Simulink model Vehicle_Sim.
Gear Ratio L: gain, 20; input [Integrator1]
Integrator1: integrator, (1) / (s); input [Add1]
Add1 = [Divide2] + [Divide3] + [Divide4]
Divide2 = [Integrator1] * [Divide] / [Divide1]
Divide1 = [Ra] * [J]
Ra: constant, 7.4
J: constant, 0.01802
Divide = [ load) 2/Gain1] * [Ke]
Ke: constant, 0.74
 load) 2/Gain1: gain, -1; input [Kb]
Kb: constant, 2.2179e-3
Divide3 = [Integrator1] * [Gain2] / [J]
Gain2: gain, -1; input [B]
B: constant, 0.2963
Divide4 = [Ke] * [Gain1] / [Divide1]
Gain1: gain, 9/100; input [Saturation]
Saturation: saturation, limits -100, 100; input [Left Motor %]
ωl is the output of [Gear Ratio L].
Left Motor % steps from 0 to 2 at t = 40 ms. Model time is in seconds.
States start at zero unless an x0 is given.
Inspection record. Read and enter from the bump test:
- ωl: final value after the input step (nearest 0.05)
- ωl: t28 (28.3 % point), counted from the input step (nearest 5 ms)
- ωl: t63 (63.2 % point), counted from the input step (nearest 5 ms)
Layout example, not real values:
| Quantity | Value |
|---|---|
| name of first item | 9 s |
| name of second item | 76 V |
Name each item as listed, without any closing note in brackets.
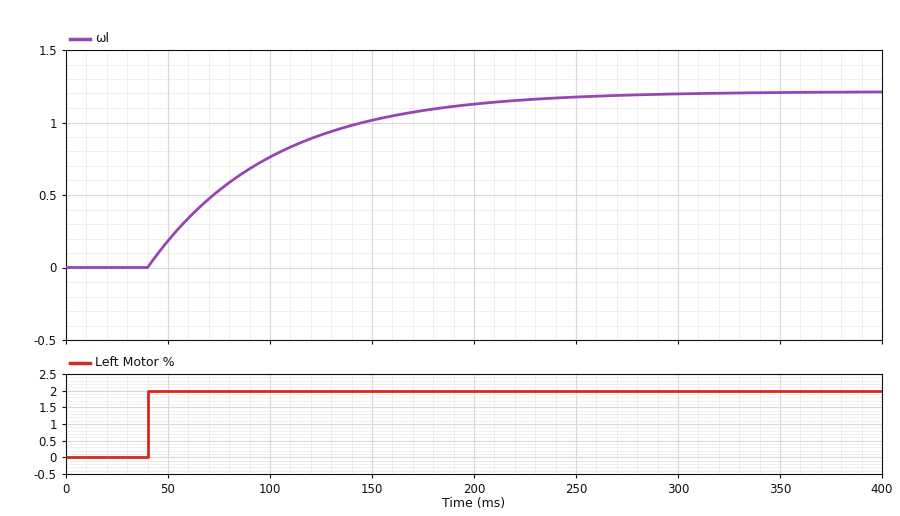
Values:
| Quantity | Value |
|---|---|
| ωl: final value after the input step | 1.20 |
| ωl: t28 (28.3 % point), counted from the input step | 20 ms |
| ωl: t63 (63.2 % point), counted from the input step | 60 ms |
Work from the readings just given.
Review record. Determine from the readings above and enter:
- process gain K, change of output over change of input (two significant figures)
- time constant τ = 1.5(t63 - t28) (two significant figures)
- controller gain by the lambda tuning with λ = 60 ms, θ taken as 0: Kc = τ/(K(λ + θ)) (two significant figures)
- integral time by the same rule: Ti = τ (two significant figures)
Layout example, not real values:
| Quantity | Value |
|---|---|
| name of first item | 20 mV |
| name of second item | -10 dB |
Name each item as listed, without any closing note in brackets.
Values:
| Quantity | Value |
|---|---|
| process gain K, change of output over change of input | 0.60 |
| time constant τ = 1.5(t63 - t28) | 60 ms |
| controller gain by the lambda tuning with λ = 60 ms, θ taken as 0: Kc = τ/(K(λ + θ)) | 1.7 |
| integral time by the same rule: Ti = τ | 60 ms |
